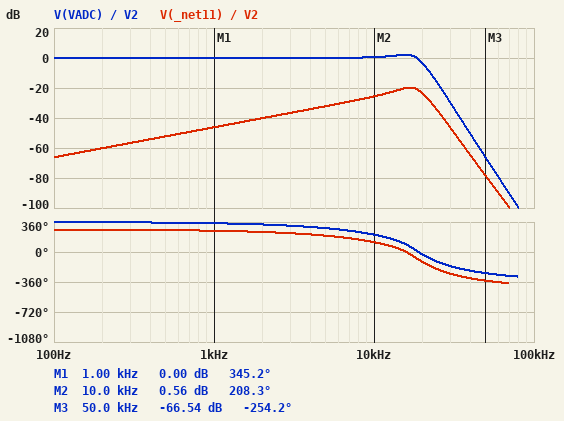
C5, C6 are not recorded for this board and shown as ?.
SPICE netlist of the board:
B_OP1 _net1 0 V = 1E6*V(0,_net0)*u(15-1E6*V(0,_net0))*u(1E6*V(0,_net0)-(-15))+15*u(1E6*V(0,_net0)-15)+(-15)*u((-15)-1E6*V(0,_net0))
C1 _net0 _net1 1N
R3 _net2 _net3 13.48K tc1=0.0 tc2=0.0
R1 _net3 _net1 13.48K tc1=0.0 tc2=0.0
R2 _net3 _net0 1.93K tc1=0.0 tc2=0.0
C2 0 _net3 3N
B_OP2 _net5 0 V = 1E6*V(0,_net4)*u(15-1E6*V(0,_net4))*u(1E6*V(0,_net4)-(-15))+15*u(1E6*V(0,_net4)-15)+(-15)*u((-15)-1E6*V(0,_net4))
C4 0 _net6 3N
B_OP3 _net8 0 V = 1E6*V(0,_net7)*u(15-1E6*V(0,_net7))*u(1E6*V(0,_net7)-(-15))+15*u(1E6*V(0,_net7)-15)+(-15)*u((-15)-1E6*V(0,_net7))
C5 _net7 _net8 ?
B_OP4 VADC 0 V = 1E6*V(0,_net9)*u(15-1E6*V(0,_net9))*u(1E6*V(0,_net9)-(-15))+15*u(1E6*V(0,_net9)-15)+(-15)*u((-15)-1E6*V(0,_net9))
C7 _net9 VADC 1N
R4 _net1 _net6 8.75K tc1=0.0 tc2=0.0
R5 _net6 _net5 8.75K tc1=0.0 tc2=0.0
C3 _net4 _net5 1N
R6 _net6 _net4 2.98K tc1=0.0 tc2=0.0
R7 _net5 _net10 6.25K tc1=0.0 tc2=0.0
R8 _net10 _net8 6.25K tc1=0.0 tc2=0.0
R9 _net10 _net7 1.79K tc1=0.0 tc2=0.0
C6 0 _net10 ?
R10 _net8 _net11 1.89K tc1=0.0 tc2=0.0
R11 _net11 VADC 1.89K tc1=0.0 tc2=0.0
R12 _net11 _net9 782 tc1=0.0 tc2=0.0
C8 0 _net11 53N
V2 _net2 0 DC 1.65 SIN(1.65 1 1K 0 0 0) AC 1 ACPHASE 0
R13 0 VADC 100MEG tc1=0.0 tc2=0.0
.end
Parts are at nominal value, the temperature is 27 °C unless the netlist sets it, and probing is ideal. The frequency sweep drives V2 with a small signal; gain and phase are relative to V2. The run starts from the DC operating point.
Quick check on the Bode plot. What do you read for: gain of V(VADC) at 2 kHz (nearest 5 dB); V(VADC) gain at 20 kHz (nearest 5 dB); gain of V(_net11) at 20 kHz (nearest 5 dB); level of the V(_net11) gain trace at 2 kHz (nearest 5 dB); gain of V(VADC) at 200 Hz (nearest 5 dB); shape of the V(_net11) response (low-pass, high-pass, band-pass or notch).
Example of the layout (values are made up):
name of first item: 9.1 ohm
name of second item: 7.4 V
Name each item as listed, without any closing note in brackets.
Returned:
gain of V(VADC) at 2 kHz: 0 dB
V(VADC) gain at 20 kHz: -5 dB
gain of V(_net11) at 20 kHz: -25 dB
level of the V(_net11) gain trace at 2 kHz: -40 dB
gain of V(VADC) at 200 Hz: 0 dB
shape of the V(_net11) response: band-pass
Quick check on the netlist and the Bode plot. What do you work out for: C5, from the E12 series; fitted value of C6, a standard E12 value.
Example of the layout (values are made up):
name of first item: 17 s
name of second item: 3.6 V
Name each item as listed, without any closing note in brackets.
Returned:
C5, from the E12 series: 560 pF
fitted value of C6, a standard E12 value: 8.2 nF
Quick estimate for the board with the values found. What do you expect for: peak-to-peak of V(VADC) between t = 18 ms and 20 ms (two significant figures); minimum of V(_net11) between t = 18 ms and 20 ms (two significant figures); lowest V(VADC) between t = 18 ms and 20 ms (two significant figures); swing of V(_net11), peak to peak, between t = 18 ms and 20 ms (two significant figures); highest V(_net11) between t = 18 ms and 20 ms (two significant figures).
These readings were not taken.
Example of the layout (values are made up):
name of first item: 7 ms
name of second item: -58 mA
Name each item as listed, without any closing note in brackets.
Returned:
peak-to-peak of V(VADC) between t = 18 ms and 20 ms: 2.0 V
minimum of V(_net11) between t = 18 ms and 20 ms: -4.9 mV
lowest V(VADC) between t = 18 ms and 20 ms: 650 mV
swing of V(_net11), peak to peak, between t = 18 ms and 20 ms: 9.8 mV
highest V(_net11) between t = 18 ms and 20 ms: 4.9 mV
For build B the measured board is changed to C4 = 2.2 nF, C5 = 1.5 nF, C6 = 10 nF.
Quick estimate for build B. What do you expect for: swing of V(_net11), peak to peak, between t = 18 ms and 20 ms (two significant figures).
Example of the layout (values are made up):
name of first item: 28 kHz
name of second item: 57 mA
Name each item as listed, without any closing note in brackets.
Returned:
swing of V(_net11), peak to peak, between t = 18 ms and 20 ms: 9.8 mV
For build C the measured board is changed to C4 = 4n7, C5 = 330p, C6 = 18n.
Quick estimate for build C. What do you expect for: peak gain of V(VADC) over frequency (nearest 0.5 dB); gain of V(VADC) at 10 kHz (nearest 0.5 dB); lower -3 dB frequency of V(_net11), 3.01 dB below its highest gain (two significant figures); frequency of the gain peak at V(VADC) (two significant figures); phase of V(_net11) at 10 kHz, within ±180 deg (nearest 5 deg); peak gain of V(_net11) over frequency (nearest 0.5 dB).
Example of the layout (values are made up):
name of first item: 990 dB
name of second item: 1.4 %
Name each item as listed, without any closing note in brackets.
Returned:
peak gain of V(VADC) over frequency: 6.5 dB
gain of V(VADC) at 10 kHz: 2.5 dB
lower -3 dB frequency of V(_net11), 3.01 dB below its highest gain: 14 kHz
frequency of the gain peak at V(VADC): 17 kHz
phase of V(_net11) at 10 kHz, within ±180 deg: 120 deg
peak gain of V(_net11) over frequency: -15.5 dB
